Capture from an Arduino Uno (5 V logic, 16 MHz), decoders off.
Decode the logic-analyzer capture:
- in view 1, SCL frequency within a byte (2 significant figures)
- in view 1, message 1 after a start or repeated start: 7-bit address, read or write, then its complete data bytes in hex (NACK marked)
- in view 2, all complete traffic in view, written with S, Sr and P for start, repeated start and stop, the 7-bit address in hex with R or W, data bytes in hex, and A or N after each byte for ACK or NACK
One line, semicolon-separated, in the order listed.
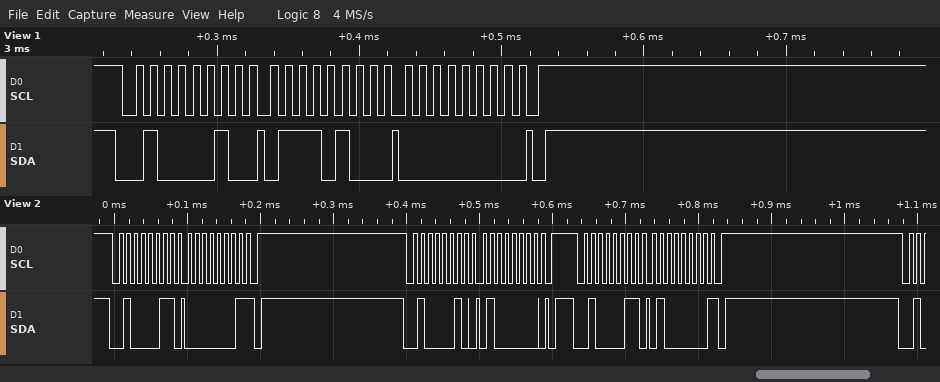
100 kHz; 0x21 write: 74 00; S 21R A 01 N P S 21W A 40 A P S 21R A 40 N P
